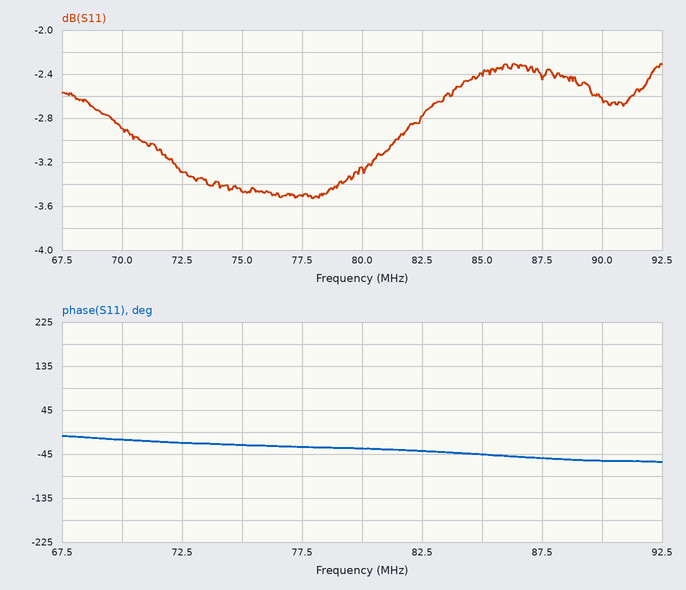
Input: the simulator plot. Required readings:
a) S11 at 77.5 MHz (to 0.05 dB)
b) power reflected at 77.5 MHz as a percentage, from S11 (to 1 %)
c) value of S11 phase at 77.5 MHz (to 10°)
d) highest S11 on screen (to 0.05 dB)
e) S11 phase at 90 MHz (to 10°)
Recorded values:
-3.50 dB
45 %
-30°
-2.30 dB
-60°
